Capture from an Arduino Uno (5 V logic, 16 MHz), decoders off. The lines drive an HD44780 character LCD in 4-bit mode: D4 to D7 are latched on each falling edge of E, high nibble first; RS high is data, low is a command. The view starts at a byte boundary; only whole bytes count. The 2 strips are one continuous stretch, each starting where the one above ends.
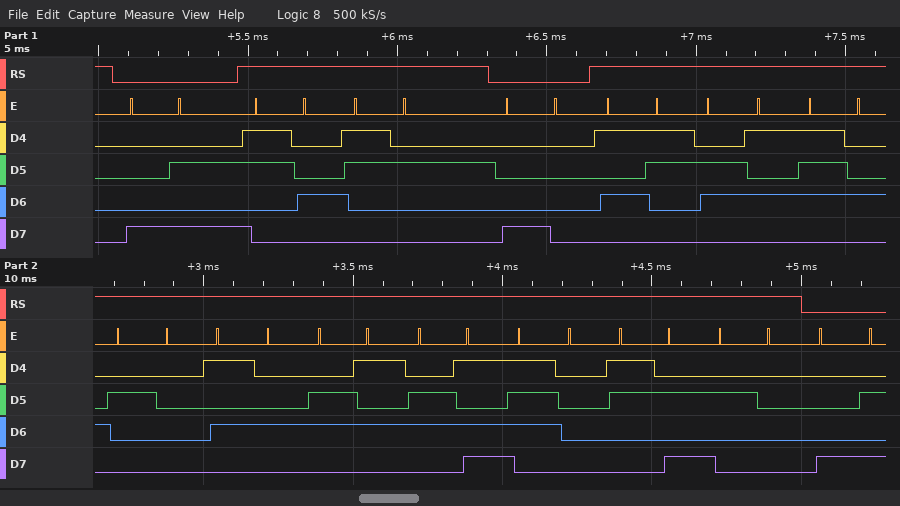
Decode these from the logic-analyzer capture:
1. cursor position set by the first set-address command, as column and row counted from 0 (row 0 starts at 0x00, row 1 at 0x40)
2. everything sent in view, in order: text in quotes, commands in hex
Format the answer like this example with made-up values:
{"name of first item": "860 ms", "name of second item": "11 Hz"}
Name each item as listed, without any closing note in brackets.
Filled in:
{"cursor position set by the first set-address command, as column and row counted from 0": "column 10, row 0", "everything sent in view, in order: text in quotes, commands in hex": "0x8A \"42\" 0x80 \"Set Temp: \" 0x8A"}
